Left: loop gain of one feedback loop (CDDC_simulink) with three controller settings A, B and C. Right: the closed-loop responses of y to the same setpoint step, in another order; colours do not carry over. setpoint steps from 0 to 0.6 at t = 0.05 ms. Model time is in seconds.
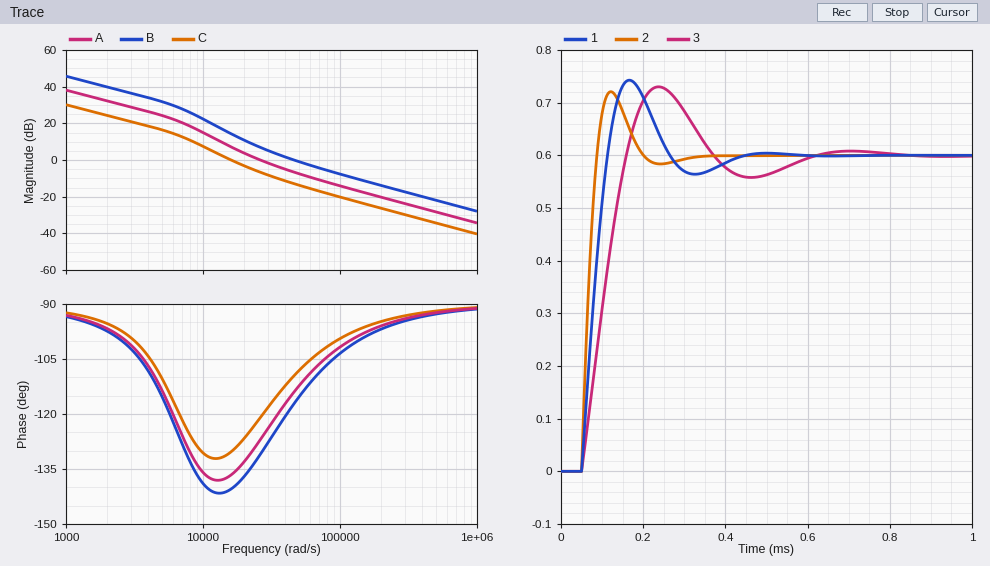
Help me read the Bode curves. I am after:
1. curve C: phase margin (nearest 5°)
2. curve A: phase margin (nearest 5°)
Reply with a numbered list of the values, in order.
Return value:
1. 50°
2. 55°
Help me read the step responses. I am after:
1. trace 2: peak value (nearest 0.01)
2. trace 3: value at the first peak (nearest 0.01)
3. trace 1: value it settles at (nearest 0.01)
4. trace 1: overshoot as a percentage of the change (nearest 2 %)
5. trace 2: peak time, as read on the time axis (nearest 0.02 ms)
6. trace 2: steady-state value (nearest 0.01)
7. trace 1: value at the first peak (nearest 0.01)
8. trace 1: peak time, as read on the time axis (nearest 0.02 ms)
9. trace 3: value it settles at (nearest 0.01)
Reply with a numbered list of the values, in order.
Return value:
1. 0.72
2. 0.73
3. 0.60
4. 24 %
5. 0.12 ms
6. 0.60
7. 0.74
8. 0.16 ms
9. 0.60
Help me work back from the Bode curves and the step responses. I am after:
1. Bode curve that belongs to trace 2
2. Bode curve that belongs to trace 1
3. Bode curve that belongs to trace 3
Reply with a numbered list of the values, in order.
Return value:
1. B
2. A
3. C
